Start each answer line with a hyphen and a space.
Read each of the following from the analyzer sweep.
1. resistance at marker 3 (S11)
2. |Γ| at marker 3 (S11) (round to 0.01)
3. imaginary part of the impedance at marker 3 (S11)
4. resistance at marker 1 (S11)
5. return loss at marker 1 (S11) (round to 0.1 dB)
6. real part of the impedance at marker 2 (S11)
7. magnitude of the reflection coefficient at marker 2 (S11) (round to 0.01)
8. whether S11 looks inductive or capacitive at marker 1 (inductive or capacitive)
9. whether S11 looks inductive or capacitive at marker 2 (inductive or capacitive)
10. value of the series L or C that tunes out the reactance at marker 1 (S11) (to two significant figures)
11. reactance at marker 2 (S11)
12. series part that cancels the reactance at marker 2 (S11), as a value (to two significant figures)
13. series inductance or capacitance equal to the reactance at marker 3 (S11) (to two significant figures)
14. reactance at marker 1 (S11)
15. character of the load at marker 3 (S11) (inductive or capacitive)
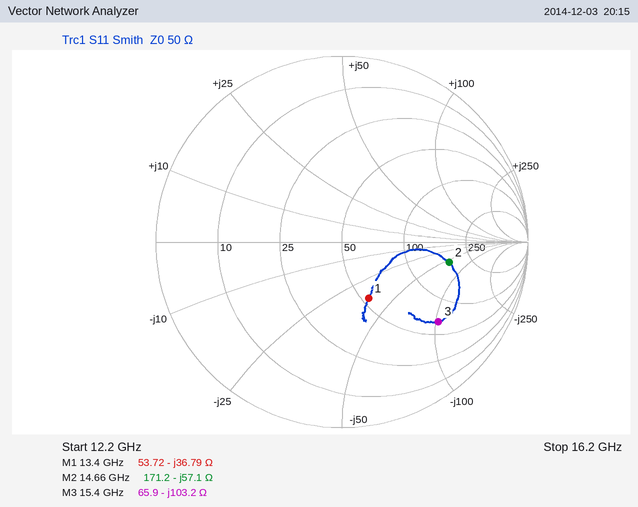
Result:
- 65.9 Ω
- 0.67
- -103.2 Ω
- 53.72 Ω
- 9.5 dB
- 171.2 Ω
- 0.59
- capacitive
- capacitive
- 440 pH
- -57.1 Ω
- 620 pH
- 100 fF
- -36.79 Ω
- capacitive
